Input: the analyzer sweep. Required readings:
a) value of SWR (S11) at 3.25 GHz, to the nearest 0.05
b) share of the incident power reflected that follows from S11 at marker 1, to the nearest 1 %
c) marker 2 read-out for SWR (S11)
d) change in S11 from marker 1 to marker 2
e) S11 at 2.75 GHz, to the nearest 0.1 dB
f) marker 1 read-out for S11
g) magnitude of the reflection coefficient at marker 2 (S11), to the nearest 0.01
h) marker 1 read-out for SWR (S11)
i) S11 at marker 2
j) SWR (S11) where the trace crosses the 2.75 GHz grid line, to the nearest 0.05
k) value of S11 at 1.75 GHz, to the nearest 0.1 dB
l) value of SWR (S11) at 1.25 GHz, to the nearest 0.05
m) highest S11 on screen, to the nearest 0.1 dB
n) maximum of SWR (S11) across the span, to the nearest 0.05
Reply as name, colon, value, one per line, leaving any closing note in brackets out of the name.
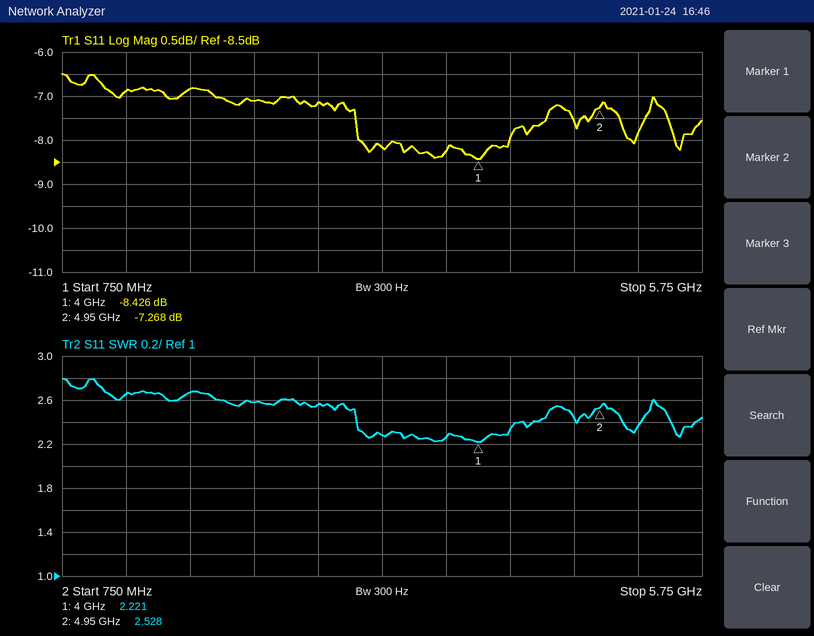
value of SWR (S11) at 3.25 GHz, to the nearest 0.05: 2.30
share of the incident power reflected that follows from S11 at marker 1, to the nearest 1 %: 14 %
marker 2 read-out for SWR: 2.528
change in S11 from marker 1 to marker 2: 1.158 dB
S11 at 2.75 GHz, to the nearest 0.1 dB: -7.2 dB
marker 1 read-out for S11: -8.426 dB
magnitude of the reflection coefficient at marker 2 (S11), to the nearest 0.01: 0.43
marker 1 read-out for SWR: 2.221
S11 at marker 2: -7.268 dB
SWR (S11) where the trace crosses the 2.75 GHz grid line, to the nearest 0.05: 2.55
value of S11 at 1.75 GHz, to the nearest 0.1 dB: -6.8 dB
value of SWR (S11) at 1.25 GHz, to the nearest 0.05: 2.65
highest S11 on screen, to the nearest 0.1 dB: -6.5 dB
maximum of SWR (S11) across the span, to the nearest 0.05: 2.80
